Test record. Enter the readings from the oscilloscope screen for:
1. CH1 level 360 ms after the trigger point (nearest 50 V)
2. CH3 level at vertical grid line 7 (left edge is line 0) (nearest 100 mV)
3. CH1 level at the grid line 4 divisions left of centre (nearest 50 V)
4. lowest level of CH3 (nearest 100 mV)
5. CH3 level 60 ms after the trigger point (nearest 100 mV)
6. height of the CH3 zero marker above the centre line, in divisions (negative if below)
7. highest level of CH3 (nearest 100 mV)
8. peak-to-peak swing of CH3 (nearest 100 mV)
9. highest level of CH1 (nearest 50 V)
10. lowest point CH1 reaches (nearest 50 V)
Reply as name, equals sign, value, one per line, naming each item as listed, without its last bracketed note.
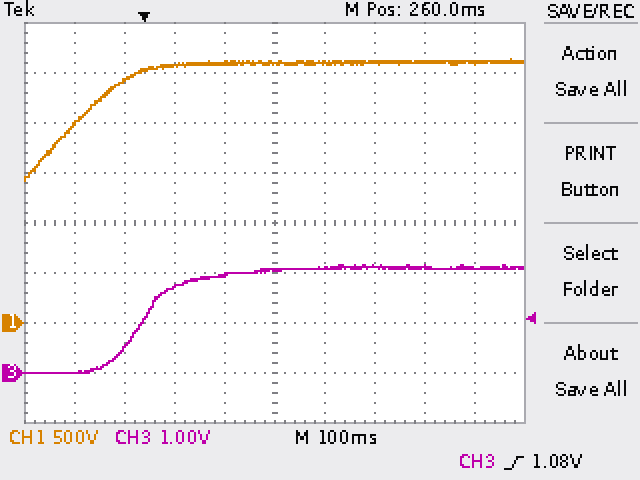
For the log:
CH1 level 360 ms after the trigger point = 2.60 kV
CH3 level at vertical grid line 7 (left edge is line 0) = 2.1 V
CH1 level at the grid line 4 divisions left of centre = 2.00 kV
lowest level of CH3 = 0.0 V
CH3 level 60 ms after the trigger point = 1.7 V
height of the CH3 zero marker above the centre line, in divisions = -3.0 div
highest level of CH3 = 2.2 V
peak-to-peak swing of CH3 = 2.2 V
highest level of CH1 = 2.65 kV
lowest point CH1 reaches = 1.40 kV
